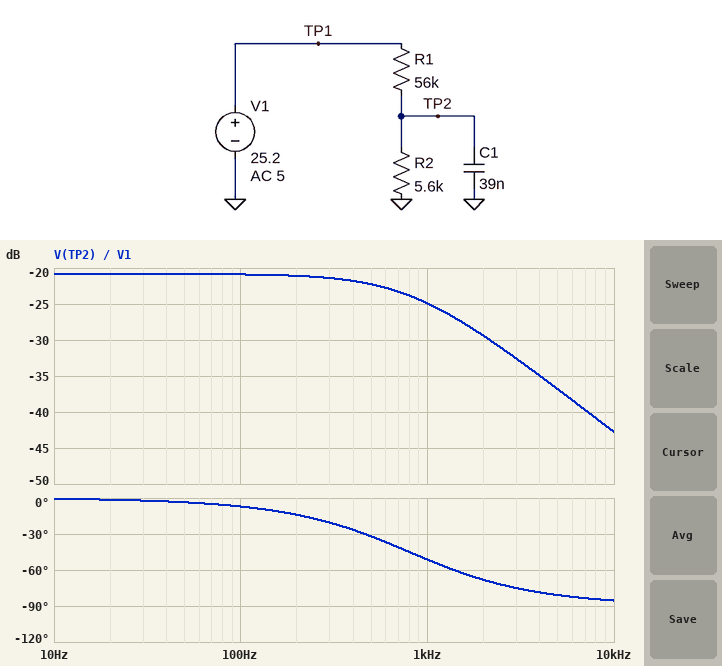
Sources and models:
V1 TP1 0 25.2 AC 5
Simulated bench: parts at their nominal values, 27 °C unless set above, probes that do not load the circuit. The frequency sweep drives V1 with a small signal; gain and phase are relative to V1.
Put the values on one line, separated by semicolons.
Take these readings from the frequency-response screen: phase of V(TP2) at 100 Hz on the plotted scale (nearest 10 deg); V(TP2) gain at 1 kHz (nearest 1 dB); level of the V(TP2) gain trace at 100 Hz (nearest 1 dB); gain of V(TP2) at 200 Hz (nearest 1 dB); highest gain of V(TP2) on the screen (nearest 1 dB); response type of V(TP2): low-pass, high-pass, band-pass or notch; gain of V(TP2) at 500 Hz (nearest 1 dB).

-10 deg; -25 dB; -21 dB; -21 dB; -21 dB; low-pass; -22 dB
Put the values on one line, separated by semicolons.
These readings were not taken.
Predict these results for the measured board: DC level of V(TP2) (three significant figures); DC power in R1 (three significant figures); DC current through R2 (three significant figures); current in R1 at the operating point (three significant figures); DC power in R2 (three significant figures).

2.29 V; 9.37 mW; 409 µA; 409 µA; 937 µW
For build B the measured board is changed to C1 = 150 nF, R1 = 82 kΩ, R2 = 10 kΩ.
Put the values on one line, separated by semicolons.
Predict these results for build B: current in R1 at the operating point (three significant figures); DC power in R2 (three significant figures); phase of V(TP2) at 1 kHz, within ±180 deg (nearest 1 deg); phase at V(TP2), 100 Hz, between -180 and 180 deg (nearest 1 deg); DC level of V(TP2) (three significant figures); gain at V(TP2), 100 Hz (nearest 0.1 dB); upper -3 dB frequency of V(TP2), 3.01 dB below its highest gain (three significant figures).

274 µA; 750 µW; -83 deg; -40 deg; 2.74 V; -21.6 dB; 119 Hz
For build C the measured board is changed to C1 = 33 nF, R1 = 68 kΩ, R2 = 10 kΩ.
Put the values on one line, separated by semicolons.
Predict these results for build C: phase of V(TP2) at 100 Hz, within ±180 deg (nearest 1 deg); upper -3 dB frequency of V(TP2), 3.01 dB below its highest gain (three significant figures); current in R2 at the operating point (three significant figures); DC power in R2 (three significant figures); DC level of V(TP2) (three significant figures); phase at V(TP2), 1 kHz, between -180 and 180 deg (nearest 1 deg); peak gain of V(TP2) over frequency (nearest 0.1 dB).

-10 deg; 553 Hz; 323 µA; 1.04 mW; 3.23 V; -61 deg; -17.8 dB
